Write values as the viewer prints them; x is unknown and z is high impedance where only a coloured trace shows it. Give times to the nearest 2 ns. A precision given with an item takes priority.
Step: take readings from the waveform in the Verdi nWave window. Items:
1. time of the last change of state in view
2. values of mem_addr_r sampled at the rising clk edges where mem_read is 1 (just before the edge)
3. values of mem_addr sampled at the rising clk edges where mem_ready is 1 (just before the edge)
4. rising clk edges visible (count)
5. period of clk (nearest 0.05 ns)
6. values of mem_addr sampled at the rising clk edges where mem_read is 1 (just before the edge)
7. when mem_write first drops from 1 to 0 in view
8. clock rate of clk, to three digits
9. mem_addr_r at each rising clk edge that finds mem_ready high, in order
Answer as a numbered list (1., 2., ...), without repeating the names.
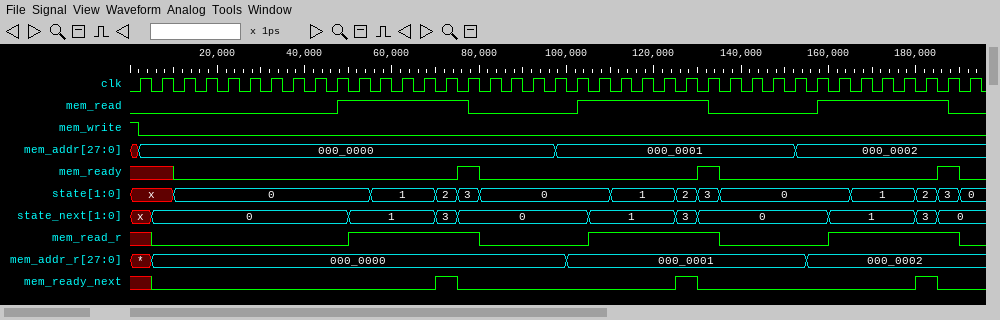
1. 190 ns
2. 000_0000, 000_0000, 000_0000, 000_0000, 000_0000, 000_0000, 000_0001, 000_0001, 000_0001, 000_0001, 000_0001, 000_0001, 000_0002, 000_0002, 000_0002, 000_0002, 000_0002, 000_0002
3. 000_0000, 000_0001, 000_0002
4. 39
5. 5 ns
6. 000_0000, 000_0000, 000_0000, 000_0000, 000_0000, 000_0000, 000_0001, 000_0001, 000_0001, 000_0001, 000_0001, 000_0001, 000_0002, 000_0002, 000_0002, 000_0002, 000_0002, 000_0002
7. 2 ns
8. 200 MHz
9. 000_0000, 000_0001, 000_0002
